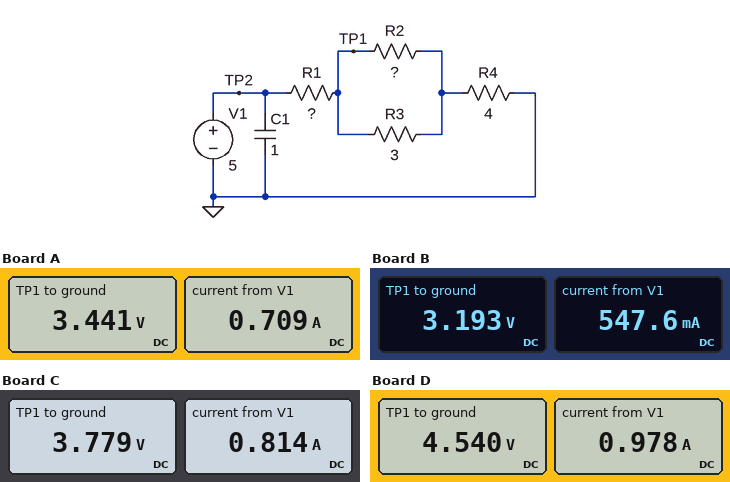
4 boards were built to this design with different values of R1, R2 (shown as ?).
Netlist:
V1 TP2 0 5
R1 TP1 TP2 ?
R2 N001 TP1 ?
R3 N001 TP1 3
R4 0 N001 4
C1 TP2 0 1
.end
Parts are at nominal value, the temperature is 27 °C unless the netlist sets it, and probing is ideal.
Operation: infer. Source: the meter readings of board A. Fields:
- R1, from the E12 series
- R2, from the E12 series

2.2 Ω
1.2 Ω
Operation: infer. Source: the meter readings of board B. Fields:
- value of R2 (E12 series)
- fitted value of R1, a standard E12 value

4.7 Ω
3.3 Ω
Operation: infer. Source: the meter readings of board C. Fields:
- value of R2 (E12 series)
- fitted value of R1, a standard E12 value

0.82 Ω
1.5 Ω
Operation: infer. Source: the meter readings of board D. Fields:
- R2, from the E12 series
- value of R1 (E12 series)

0.82 Ω
0.47 Ω
